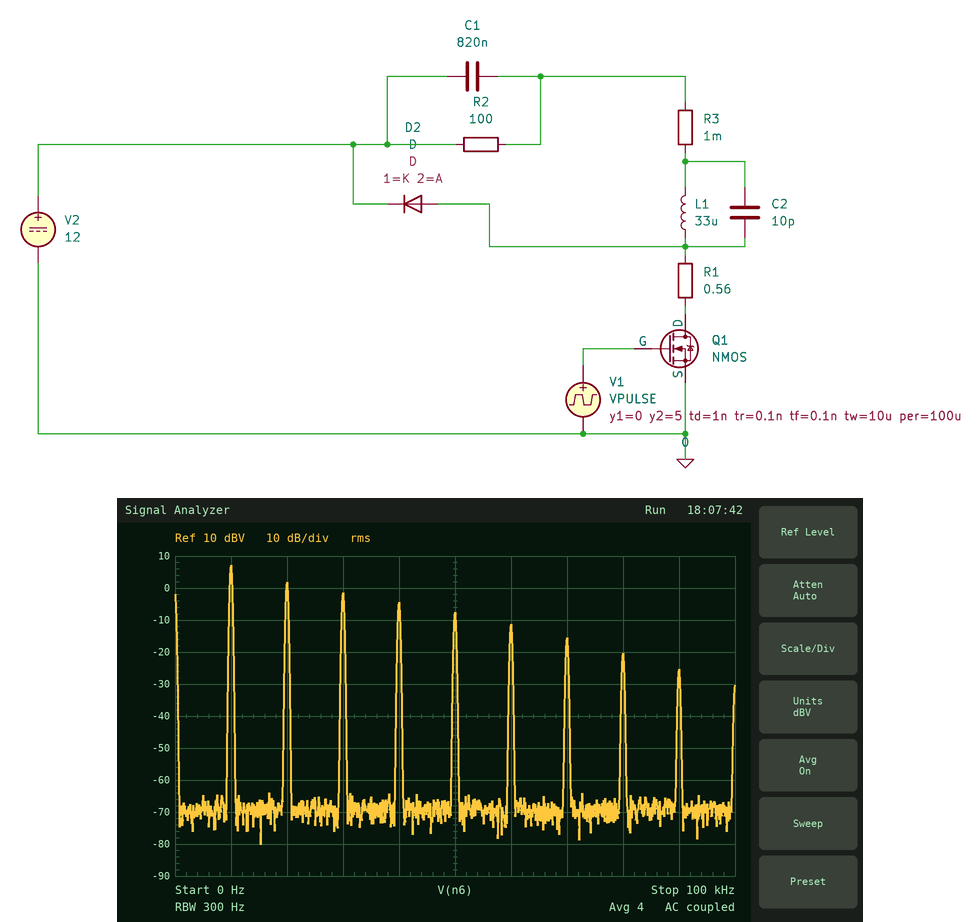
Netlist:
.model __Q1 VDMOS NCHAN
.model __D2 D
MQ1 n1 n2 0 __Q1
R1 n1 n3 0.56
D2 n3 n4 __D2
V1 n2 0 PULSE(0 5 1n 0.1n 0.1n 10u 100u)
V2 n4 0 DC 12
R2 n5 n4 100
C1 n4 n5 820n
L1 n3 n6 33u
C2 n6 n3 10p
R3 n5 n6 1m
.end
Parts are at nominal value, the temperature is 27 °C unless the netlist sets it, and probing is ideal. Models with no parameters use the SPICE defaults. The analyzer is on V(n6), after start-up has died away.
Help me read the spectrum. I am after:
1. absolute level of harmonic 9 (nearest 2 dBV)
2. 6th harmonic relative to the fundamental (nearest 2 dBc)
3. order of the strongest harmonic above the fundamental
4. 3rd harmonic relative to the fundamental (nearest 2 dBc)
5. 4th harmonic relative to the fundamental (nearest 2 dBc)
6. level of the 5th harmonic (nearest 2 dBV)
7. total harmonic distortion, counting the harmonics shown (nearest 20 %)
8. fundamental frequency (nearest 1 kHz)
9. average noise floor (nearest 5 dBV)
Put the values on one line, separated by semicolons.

-26 dBV; -18 dBc; 2; -8 dBc; -12 dBc; -8 dBV; 80 %; 10 kHz; -70 dBV
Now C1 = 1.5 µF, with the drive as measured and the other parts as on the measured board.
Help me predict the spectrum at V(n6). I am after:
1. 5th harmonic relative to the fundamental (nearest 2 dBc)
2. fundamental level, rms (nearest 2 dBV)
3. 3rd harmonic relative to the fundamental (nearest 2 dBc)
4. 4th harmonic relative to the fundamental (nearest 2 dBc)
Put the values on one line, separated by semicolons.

-18 dBc; 2 dBV; -10 dBc; -14 dBc
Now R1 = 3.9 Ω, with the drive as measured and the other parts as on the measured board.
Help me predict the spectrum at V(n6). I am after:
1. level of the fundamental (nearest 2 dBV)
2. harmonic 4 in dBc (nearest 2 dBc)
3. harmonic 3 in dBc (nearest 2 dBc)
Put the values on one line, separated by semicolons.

6 dBV; -14 dBc; -10 dBc
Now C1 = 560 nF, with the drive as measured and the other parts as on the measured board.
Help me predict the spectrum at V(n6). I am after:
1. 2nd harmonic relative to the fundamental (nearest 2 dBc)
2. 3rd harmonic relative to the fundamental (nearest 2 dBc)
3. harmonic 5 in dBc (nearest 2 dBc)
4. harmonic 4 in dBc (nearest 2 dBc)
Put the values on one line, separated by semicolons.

-4 dBc; -6 dBc; -12 dBc; -8 dBc
